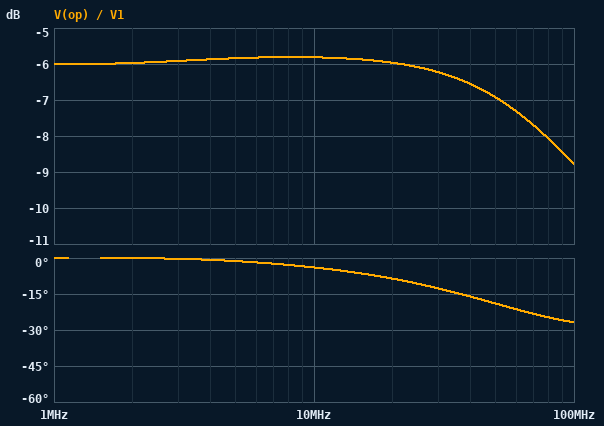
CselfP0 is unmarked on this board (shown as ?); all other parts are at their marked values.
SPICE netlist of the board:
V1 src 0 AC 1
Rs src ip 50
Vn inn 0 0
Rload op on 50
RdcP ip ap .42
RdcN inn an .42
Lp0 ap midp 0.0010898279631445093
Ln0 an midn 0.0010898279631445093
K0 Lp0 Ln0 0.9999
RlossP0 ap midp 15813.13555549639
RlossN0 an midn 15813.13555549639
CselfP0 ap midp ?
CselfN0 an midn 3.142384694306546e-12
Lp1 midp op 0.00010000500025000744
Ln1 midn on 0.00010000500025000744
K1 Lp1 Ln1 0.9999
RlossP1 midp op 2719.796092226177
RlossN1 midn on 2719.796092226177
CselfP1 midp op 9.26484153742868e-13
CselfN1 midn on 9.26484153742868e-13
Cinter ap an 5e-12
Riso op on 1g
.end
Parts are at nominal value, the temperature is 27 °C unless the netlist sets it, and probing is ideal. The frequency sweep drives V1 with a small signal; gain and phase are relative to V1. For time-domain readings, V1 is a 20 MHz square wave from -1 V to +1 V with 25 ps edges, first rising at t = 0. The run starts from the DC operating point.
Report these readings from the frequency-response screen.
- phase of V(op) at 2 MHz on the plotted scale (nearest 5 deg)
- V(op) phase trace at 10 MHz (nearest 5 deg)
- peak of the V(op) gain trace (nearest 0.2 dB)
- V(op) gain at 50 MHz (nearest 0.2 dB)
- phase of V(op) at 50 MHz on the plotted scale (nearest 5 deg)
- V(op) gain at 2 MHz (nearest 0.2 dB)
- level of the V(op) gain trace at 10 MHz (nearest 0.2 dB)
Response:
0 deg
-5 deg
-5.8 dB
-7.0 dB
-20 deg
-6.0 dB
-5.8 dB
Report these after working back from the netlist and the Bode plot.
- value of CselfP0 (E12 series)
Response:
1 pF
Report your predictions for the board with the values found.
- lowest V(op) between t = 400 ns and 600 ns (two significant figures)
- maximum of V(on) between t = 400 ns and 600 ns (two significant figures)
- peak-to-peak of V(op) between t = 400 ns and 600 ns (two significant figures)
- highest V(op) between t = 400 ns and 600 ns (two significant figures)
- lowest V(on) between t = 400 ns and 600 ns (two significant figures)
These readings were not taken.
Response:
-520 mV
480 mV
1.0 V
520 mV
-480 mV
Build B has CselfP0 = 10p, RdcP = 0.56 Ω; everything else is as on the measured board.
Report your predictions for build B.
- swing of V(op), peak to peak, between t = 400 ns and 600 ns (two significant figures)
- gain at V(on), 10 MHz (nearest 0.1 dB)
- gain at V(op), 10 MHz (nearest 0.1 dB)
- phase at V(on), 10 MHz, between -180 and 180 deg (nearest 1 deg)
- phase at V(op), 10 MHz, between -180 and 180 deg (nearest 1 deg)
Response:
1.8 V
-19.3 dB
-6.0 dB
82 deg
4 deg
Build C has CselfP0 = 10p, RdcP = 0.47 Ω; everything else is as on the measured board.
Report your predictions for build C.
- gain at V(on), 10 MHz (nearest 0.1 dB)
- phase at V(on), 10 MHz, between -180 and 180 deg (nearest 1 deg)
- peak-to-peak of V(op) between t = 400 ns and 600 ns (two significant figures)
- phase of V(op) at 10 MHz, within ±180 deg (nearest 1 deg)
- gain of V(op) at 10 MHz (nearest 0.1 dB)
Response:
-19.3 dB
82 deg
1.8 V
4 deg
-6.0 dB
